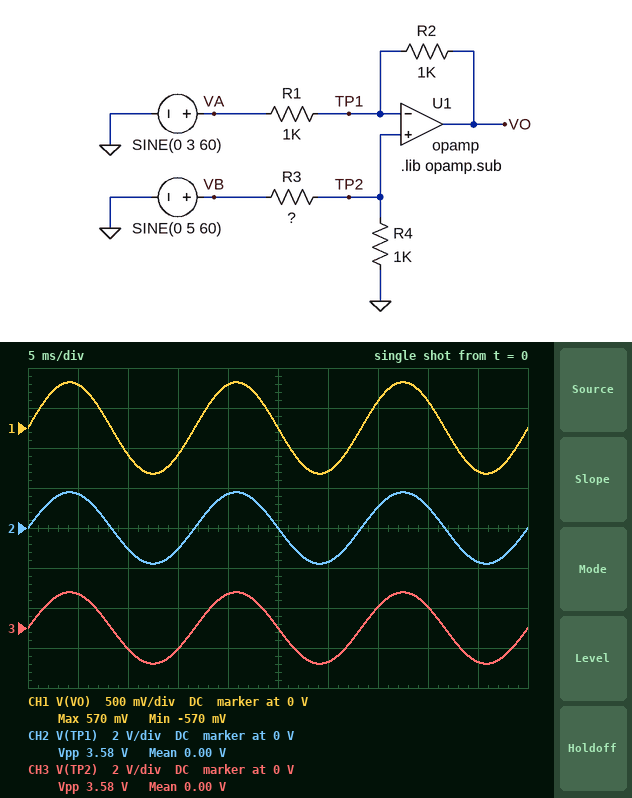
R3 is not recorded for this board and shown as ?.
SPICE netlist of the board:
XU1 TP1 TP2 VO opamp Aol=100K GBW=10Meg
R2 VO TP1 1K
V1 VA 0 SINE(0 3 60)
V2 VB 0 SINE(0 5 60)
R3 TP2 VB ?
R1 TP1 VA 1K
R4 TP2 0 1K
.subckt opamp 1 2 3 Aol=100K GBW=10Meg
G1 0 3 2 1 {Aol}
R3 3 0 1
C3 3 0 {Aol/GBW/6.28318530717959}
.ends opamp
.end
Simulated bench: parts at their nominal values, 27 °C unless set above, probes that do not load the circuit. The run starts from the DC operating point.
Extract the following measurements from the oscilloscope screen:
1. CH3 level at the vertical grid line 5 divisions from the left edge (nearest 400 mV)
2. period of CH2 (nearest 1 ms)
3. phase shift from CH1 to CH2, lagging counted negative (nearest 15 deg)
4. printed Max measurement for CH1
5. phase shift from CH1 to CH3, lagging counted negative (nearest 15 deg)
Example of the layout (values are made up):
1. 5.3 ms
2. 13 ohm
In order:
1. 0 V
2. 17 ms
3. 0 deg
4. 570 mV
5. 0 deg
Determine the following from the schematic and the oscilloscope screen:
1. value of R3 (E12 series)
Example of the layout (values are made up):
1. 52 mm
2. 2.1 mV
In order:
1. 1.8 kΩ
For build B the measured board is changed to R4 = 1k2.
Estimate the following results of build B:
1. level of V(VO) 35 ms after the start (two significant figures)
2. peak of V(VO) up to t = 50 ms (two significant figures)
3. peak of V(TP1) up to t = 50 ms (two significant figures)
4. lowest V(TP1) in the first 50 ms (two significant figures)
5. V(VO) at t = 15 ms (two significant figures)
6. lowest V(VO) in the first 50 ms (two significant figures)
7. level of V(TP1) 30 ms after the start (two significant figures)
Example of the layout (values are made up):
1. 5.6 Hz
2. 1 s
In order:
1. 590 mV
2. 1.0 V
3. 2.0 V
4. -2.0 V
5. -590 mV
6. -1.0 V
7. -1.9 V
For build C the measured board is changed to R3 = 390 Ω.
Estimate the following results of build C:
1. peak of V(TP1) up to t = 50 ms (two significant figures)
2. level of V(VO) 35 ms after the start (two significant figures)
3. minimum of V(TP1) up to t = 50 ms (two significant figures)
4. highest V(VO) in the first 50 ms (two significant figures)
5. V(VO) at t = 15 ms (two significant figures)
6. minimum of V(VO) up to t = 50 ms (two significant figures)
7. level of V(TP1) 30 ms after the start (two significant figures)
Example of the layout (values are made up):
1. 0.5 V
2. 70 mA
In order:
1. 3.6 V
2. 2.5 V
3. -3.6 V
4. 4.2 V
5. -2.5 V
6. -4.2 V
7. -3.4 V
